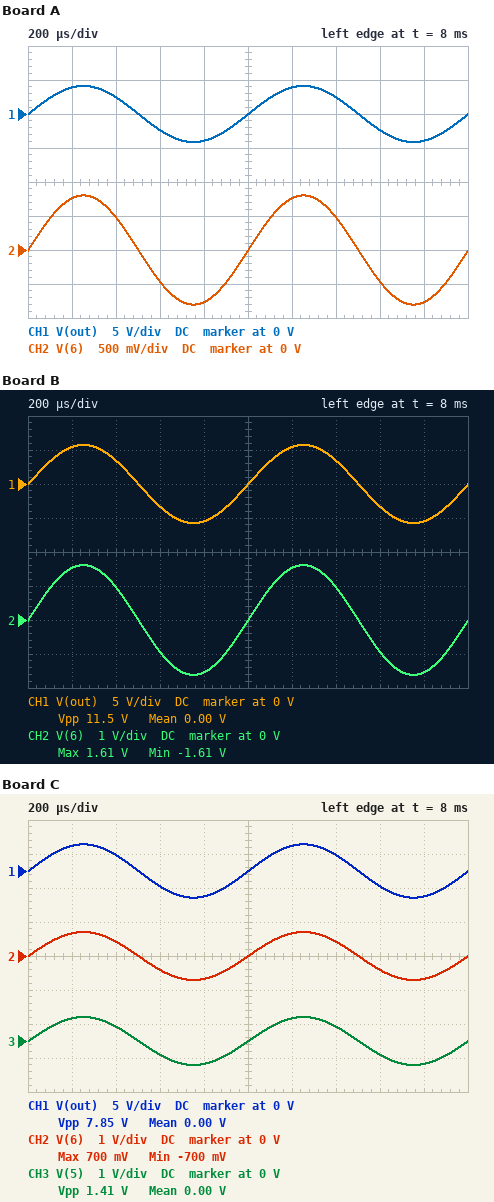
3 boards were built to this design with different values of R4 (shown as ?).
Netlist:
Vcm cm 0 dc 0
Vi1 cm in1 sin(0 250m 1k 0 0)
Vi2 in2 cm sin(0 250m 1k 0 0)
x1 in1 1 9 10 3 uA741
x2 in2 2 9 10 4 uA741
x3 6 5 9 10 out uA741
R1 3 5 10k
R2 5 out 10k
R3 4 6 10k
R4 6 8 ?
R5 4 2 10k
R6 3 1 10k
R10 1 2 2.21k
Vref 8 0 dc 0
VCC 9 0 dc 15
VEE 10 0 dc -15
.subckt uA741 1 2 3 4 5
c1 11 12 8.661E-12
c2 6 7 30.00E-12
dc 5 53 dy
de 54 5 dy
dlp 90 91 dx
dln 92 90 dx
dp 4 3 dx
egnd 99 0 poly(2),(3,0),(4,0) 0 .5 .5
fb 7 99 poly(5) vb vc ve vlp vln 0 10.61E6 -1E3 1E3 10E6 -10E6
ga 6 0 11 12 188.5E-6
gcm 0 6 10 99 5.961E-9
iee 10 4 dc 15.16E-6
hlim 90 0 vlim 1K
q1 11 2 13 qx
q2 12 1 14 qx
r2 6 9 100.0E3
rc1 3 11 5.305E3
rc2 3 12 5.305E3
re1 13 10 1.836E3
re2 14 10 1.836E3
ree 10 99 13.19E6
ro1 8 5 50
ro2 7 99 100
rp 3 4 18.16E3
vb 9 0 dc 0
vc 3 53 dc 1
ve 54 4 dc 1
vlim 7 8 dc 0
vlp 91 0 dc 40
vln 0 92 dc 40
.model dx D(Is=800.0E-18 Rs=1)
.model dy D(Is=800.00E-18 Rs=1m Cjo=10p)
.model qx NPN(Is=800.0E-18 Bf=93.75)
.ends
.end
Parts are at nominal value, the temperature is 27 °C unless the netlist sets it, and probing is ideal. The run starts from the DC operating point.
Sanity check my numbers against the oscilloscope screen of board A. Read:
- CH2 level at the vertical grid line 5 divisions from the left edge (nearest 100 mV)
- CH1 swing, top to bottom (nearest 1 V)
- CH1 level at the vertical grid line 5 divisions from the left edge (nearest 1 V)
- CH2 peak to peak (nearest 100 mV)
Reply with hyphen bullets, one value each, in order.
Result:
- 0 V
- 8 V
- 0 V
- 1.6 V
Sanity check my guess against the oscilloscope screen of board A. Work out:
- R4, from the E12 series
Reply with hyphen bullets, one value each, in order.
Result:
- 4.7 kΩ
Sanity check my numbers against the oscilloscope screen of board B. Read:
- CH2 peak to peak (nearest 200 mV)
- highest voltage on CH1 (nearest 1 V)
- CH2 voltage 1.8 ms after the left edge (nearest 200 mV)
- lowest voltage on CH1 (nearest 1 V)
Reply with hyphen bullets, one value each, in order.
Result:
- 3.2 V
- 6 V
- -1.6 V
- -6 V
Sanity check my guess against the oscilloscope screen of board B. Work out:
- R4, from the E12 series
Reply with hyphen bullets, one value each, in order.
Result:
- 18 kΩ
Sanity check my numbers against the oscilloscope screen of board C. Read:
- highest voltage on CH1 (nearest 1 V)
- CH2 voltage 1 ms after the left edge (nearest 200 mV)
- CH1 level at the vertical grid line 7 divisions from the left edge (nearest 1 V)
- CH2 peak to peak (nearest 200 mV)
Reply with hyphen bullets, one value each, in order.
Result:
- 4 V
- 0 V
- 2 V
- 1.4 V
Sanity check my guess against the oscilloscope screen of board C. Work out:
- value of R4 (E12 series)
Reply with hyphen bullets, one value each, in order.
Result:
- 3.9 kΩ
